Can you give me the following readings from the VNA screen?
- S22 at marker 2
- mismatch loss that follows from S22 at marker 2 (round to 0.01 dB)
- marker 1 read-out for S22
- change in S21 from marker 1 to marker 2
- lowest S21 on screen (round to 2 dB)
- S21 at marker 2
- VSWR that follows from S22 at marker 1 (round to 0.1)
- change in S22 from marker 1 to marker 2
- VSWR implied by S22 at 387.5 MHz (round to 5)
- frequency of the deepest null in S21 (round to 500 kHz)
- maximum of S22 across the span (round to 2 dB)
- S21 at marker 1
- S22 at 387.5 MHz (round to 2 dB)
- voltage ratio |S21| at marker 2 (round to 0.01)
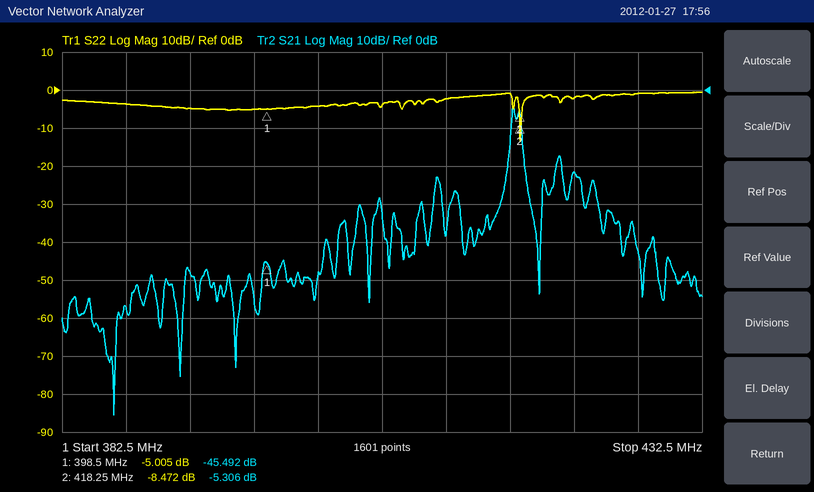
-8.472 dB
0.67 dB
-5.005 dB
40.186 dB
-86 dB
-5.306 dB
3.6
-3.467 dB
5
386.5 MHz
0 dB
-45.492 dB
-4 dB
0.54
